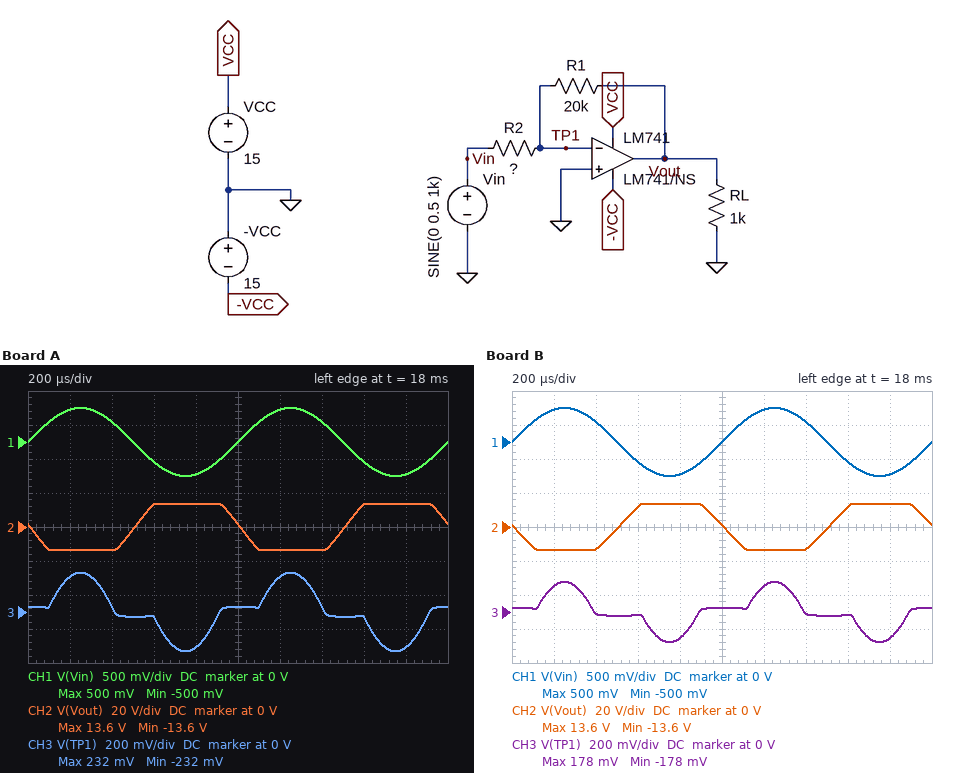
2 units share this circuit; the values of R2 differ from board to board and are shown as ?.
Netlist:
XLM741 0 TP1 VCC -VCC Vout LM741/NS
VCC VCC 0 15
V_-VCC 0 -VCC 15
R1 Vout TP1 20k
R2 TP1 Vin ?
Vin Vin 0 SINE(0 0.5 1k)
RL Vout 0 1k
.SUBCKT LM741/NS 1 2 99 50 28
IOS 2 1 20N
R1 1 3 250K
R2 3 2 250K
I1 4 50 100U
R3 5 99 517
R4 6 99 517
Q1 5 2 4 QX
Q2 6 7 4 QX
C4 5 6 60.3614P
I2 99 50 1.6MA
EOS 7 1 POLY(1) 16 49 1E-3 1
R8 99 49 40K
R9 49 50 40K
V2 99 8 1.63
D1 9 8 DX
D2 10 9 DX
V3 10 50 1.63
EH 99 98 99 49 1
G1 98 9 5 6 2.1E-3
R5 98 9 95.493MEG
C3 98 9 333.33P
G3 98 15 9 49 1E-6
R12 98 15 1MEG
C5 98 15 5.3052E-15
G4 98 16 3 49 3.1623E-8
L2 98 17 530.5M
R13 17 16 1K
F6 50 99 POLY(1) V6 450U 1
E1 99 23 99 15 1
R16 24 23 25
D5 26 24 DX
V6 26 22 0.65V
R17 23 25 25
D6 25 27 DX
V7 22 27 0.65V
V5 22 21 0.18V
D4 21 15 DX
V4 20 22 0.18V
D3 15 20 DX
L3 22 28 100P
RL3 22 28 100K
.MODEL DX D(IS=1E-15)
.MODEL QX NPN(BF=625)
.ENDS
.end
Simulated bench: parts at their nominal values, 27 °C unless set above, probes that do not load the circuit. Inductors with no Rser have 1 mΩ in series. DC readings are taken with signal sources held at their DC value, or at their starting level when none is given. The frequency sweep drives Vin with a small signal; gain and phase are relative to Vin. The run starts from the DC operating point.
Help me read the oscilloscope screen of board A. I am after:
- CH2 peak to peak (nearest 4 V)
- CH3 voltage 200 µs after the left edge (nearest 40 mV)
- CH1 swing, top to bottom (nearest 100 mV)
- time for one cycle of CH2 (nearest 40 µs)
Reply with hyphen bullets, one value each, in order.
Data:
- 28 V
- 200 mV
- 1.0 V
- 1.00 ms
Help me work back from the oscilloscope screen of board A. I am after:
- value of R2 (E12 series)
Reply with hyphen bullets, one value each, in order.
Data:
- 390 Ω
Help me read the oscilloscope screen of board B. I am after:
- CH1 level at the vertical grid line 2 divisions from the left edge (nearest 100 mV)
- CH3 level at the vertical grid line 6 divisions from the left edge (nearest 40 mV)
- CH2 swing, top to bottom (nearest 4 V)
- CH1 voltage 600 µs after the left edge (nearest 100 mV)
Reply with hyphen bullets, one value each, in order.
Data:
- 300 mV
- 160 mV
- 28 V
- -300 mV
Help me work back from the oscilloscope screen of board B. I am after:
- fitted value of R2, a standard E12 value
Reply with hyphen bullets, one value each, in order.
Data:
- 470 Ω
